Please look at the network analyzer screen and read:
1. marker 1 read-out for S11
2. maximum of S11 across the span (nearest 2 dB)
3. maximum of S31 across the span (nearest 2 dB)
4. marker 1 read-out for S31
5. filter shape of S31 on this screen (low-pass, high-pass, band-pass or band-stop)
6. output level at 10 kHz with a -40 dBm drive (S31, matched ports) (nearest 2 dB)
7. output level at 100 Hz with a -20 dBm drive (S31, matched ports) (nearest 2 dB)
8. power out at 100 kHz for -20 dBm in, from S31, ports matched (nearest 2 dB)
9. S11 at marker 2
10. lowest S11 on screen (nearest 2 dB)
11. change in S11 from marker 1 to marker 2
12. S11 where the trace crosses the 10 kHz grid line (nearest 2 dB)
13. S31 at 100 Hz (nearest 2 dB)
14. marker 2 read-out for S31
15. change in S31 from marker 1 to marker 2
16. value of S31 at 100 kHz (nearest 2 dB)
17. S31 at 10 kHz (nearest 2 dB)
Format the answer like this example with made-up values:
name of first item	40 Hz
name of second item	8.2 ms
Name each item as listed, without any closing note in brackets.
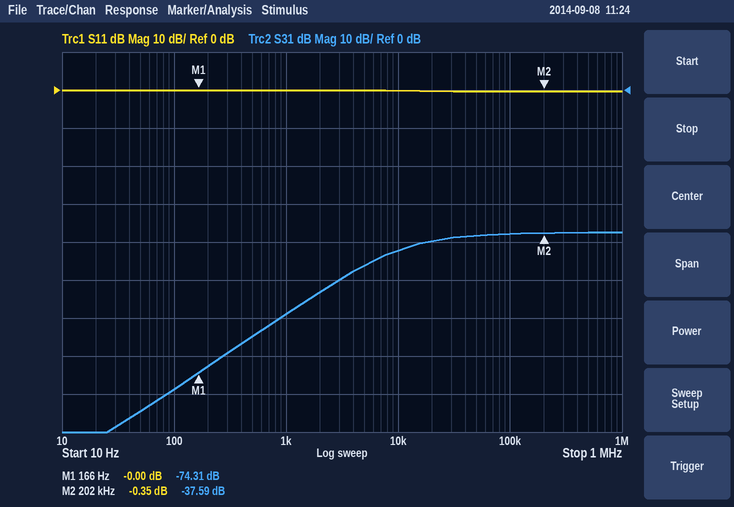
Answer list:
marker 1 read-out for S11	-0.00 dB
maximum of S11 across the span	0 dB
maximum of S31 across the span	-38 dB
marker 1 read-out for S31	-74.31 dB
filter shape of S31 on this screen	high-pass
output level at 10 kHz with a -40 dBm drive (S31, matched ports)	-82 dBm
output level at 100 Hz with a -20 dBm drive (S31, matched ports)	-98 dBm
power out at 100 kHz for -20 dBm in, from S31, ports matched	-58 dBm
S11 at marker 2	-0.35 dB
lowest S11 on screen	0 dB
change in S11 from marker 1 to marker 2	-0.35 dB
S11 where the trace crosses the 10 kHz grid line	0 dB
S31 at 100 Hz	-78 dB
marker 2 read-out for S31	-37.59 dB
change in S31 from marker 1 to marker 2	36.72 dB
value of S31 at 100 kHz	-38 dB
S31 at 10 kHz	-42 dB
